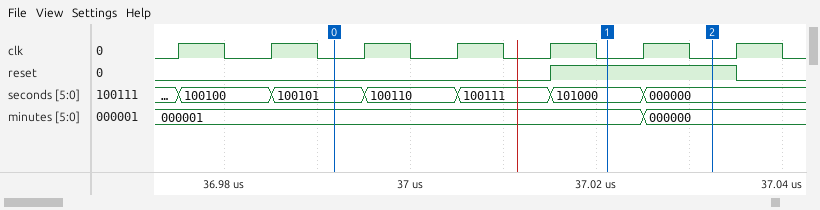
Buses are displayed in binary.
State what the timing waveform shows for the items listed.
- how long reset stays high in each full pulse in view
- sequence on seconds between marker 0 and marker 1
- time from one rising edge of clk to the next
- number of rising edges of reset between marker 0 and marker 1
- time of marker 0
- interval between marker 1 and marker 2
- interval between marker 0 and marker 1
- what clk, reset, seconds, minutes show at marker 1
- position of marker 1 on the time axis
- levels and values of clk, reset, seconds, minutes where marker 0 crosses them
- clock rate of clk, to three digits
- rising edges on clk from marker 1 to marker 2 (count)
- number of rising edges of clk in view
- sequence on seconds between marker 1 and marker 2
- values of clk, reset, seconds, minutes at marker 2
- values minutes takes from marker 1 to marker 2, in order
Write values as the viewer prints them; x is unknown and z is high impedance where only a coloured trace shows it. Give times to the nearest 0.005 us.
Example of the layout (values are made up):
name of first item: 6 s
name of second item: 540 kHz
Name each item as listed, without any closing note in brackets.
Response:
how long reset stays high in each full pulse in view: 0.02 us
sequence on seconds between marker 0 and marker 1: 100101, 100110, 100111, 101000
time from one rising edge of clk to the next: 0.01 us
number of rising edges of reset between marker 0 and marker 1: 1
time of marker 0: 36.99 us
interval between marker 1 and marker 2: 0.01 us
interval between marker 0 and marker 1: 0.03 us
what clk, reset, seconds, minutes show at marker 1: clk=0, reset=1, seconds=101000, minutes=000001
position of marker 1 on the time axis: 37.02 us
levels and values of clk, reset, seconds, minutes where marker 0 crosses them: clk=0, reset=0, seconds=100101, minutes=000001
clock rate of clk, to three digits: 100 MHz
rising edges on clk from marker 1 to marker 2: 1
number of rising edges of clk in view: 7
sequence on seconds between marker 1 and marker 2: 101000, 000000
values of clk, reset, seconds, minutes at marker 2: clk=0, reset=1, seconds=000000, minutes=000000
values minutes takes from marker 1 to marker 2, in order: 000001, 000000
